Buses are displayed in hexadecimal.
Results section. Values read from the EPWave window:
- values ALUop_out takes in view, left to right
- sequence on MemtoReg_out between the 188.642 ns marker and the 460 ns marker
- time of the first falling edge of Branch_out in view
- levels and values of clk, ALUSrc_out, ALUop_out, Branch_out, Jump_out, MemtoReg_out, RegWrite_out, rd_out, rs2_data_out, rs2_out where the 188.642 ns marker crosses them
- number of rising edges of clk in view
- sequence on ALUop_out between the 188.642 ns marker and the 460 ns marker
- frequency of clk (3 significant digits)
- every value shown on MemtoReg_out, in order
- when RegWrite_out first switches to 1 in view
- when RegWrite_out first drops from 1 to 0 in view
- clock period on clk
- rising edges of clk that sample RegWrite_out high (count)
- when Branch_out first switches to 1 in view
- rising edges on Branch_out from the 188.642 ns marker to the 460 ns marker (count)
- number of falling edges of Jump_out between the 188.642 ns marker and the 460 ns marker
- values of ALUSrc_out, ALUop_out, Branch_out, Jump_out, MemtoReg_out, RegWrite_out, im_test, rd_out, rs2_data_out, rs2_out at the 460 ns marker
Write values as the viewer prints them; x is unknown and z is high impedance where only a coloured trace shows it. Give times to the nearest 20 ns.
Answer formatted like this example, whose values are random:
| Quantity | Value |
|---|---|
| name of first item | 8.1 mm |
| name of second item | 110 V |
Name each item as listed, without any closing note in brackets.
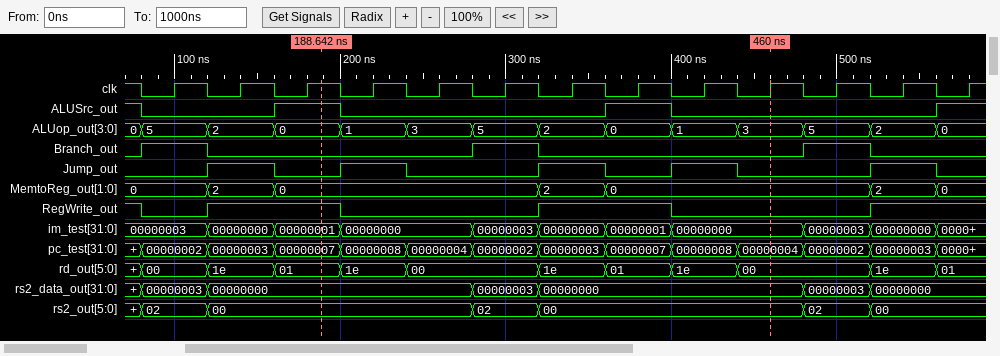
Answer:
| Quantity | Value |
|---|---|
| values ALUop_out takes in view, left to right | 0, 5, 2, 0, 1, 3, 5, 2, 0, 1, 3, 5, 2, 0 |
| sequence on MemtoReg_out between the 188.642 ns marker and the 460 ns marker | 0, 2, 0 |
| time of the first falling edge of Branch_out in view | 120 ns |
| levels and values of clk, ALUSrc_out, ALUop_out, Branch_out, Jump_out, MemtoReg_out, RegWrite_out, rd_out, rs2_data_out, rs2_out where the 188.642 ns marker crosses them | clk=1, ALUSrc_out=1, ALUop_out=0, Branch_out=0, Jump_out=0, MemtoReg_out=0, RegWrite_out=1, rd_out=01, rs2_data_out=00000000, rs2_out=00 |
| number of rising edges of clk in view | 13 |
| sequence on ALUop_out between the 188.642 ns marker and the 460 ns marker | 0, 1, 3, 5, 2, 0, 1, 3 |
| frequency of clk | 25.0 MHz |
| every value shown on MemtoReg_out, in order | 0, 2, 0, 2, 0, 2, 0 |
| when RegWrite_out first switches to 1 in view | 120 ns |
| when RegWrite_out first drops from 1 to 0 in view | 80 ns |
| clock period on clk | 40 ns |
| rising edges of clk that sample RegWrite_out high | 6 |
| when Branch_out first switches to 1 in view | 80 ns |
| rising edges on Branch_out from the 188.642 ns marker to the 460 ns marker | 1 |
| number of falling edges of Jump_out between the 188.642 ns marker and the 460 ns marker | 3 |
| values of ALUSrc_out, ALUop_out, Branch_out, Jump_out, MemtoReg_out, RegWrite_out, im_test, rd_out, rs2_data_out, rs2_out at the 460 ns marker | ALUSrc_out=0, ALUop_out=3, Branch_out=0, Jump_out=0, MemtoReg_out=0, RegWrite_out=0, im_test=00000000, rd_out=00, rs2_data_out=00000000, rs2_out=00 |
